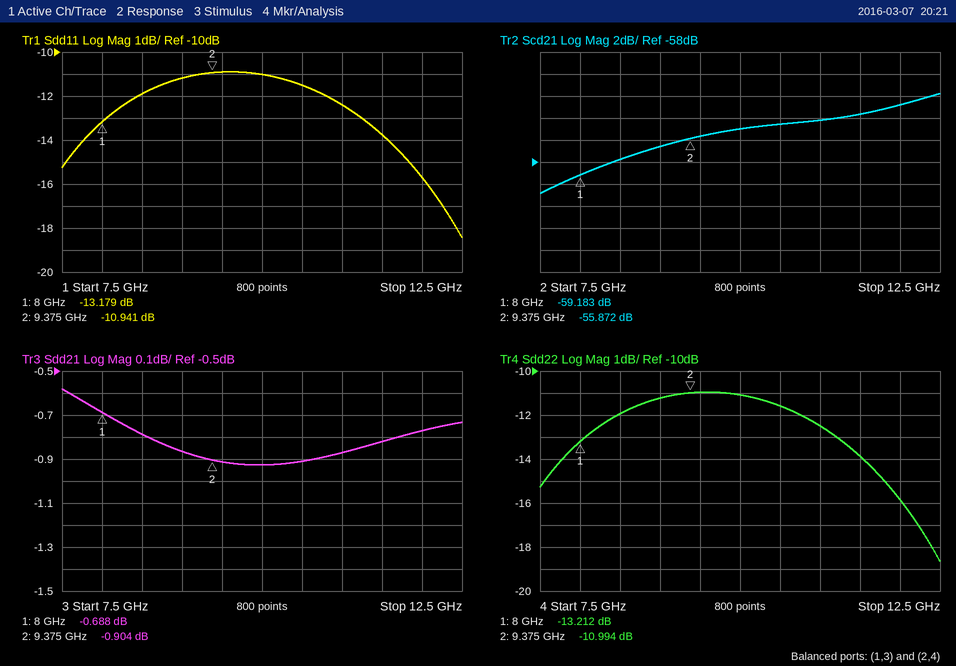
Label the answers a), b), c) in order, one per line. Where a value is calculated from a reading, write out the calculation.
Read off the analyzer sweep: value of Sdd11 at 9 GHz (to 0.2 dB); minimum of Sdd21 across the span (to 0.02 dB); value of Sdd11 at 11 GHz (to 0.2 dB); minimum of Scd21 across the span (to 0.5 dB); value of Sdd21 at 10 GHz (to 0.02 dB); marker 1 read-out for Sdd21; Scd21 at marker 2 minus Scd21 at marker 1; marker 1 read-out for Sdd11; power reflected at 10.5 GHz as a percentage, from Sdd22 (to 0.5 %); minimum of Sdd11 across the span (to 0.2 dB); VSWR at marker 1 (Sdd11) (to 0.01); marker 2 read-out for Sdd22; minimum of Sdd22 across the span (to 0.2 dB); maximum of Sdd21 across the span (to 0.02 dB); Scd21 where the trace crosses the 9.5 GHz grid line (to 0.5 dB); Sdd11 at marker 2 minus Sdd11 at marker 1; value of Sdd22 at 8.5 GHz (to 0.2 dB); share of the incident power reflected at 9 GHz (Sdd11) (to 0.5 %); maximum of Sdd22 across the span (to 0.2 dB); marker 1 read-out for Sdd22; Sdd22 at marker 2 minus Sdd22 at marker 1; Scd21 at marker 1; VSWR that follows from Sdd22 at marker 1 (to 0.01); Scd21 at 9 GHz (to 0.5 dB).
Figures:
a) -11.2 dB
b) -0.92 dB
c) -12.4 dB
d) -61.0 dB
e) -0.92 dB
f) -0.688 dB
g) -55.872 − (-59.183) = 3.311 dB
h) -13.179 dB
i) 10^(-11.6/10) ≈ 6.92 %, so 7.0 % to the nearest 0.5 %
j) -18.4 dB
k) (1 + 0.2193)/(1 − 0.2193) ≈ 1.56
l) -10.994 dB
m) -18.6 dB
n) -0.58 dB
o) -55.5 dB
p) -10.941 − (-13.179) = 2.238 dB
q) -12.0 dB
r) 10^(-11.2/10) ≈ 7.59 %, so 7.5 % to the nearest 0.5 %
s) -11.0 dB
t) -13.212 dB
u) -10.994 − (-13.212) = 2.218 dB
v) -59.183 dB
w) (1 + 0.2185)/(1 − 0.2185) ≈ 1.56
x) -56.5 dB
